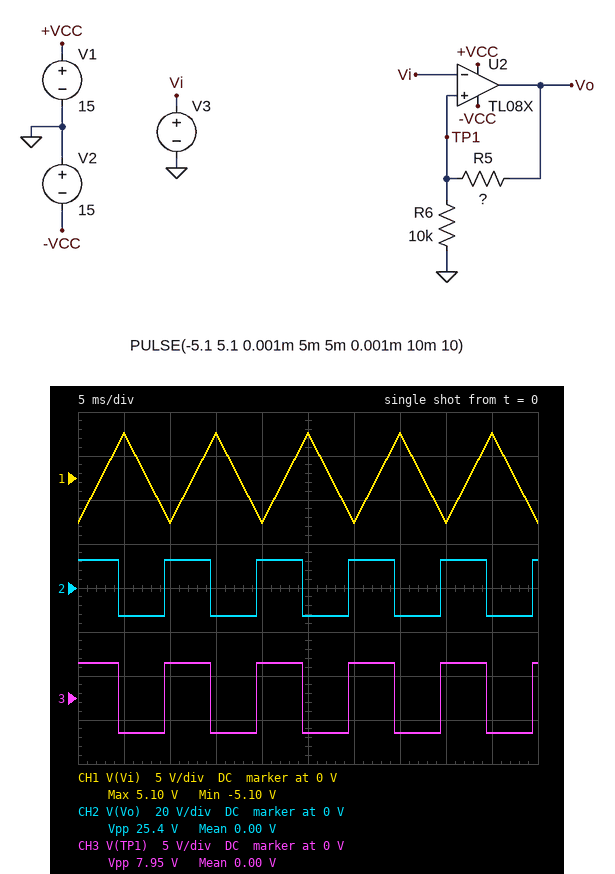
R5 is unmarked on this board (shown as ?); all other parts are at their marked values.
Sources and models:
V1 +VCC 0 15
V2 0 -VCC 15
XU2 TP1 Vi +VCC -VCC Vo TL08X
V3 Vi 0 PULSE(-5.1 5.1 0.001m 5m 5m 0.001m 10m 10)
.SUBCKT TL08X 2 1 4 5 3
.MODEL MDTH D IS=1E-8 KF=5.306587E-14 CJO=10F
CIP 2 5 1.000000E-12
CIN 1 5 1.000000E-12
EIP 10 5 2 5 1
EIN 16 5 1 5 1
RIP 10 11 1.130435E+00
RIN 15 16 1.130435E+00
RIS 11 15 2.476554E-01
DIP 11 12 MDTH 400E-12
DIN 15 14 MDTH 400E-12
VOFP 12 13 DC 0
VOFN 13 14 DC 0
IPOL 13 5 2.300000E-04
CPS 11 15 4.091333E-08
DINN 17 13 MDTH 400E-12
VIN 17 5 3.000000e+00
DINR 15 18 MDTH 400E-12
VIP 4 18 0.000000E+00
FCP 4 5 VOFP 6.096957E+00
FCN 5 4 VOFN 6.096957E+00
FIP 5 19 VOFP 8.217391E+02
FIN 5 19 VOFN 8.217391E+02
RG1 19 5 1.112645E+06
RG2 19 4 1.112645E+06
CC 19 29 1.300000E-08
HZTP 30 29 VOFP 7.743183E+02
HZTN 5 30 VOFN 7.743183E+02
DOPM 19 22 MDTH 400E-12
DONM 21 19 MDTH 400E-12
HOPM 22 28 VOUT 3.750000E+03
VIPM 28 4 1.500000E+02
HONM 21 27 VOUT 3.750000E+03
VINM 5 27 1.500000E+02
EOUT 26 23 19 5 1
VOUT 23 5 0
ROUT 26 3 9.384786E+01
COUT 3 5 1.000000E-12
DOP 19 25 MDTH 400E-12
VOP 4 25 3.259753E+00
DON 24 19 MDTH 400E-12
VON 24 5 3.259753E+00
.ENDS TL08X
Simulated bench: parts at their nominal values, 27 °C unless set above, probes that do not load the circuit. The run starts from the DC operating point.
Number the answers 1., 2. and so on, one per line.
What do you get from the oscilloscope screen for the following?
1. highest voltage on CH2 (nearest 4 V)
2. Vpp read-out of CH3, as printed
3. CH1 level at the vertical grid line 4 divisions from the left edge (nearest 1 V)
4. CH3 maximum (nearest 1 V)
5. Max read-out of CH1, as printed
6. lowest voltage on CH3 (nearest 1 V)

1. 12 V
2. 7.95 V
3. -5 V
4. 4 V
5. 5.10 V
6. -4 V
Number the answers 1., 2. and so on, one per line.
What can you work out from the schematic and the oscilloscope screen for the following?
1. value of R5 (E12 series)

1. 22 kΩ
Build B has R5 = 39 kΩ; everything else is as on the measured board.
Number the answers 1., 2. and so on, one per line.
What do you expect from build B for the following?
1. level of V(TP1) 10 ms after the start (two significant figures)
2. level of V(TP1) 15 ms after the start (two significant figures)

1. 2.6 V
2. -2.6 V
